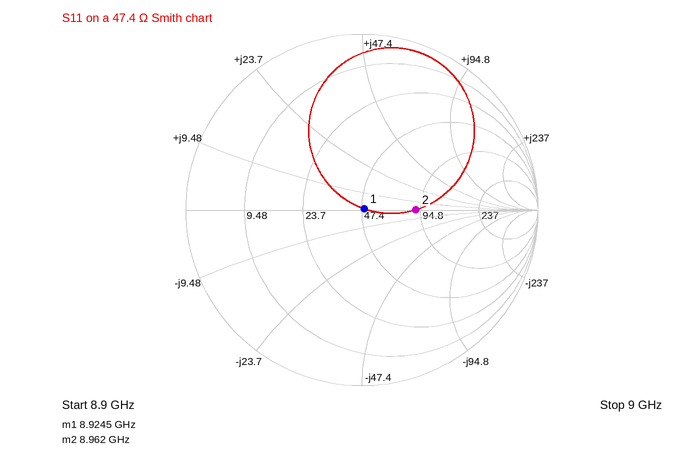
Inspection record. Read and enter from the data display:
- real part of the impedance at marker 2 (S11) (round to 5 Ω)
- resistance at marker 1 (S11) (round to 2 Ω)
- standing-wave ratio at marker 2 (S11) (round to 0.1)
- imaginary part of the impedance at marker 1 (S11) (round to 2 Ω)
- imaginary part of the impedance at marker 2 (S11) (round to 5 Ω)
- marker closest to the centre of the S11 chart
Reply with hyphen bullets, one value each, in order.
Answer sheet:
- 90 Ω
- 48 Ω
- 1.9
- 0 Ω
- 0 Ω
- marker 1
